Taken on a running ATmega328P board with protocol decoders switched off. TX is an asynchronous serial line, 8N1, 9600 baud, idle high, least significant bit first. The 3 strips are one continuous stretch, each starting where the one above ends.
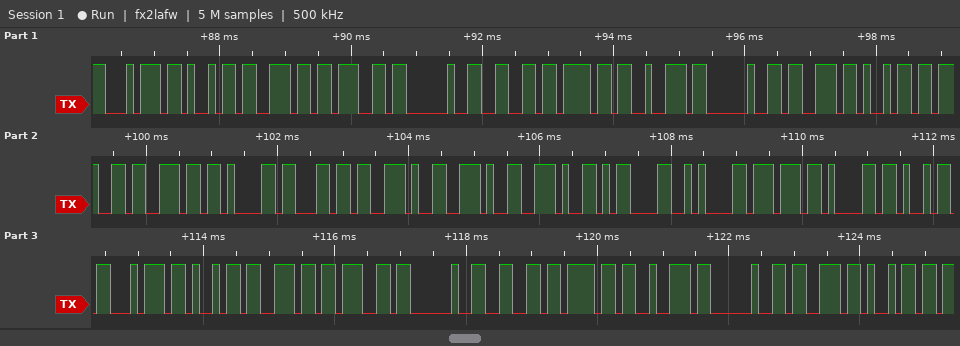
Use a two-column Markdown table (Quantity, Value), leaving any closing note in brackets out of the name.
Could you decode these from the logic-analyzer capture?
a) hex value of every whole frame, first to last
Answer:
| Quantity | Value |
|---|---|
| hex value of every whole frame, first to last | 74 69 6E 67 20 66 6F 72 20 73 69 67 6E 61 6C 2E 2E 2E 0D 0A 77 61 69 74 69 6E 67 20 66 6F 72 20 73 69 |
